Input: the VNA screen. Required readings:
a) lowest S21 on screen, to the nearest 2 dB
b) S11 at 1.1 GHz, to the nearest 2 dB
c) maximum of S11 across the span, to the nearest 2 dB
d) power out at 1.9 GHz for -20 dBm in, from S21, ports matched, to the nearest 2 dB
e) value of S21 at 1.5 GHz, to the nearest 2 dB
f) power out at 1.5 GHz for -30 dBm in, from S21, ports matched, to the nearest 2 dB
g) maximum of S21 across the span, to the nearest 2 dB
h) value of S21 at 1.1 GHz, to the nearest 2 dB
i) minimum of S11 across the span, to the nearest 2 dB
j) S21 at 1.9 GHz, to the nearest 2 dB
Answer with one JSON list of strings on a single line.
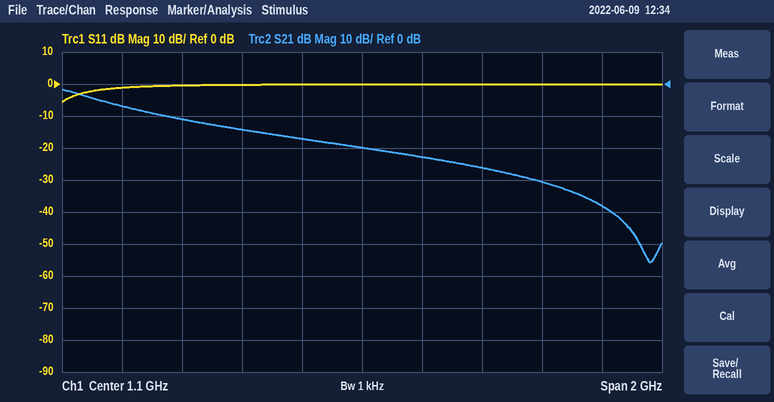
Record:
["-56 dB", "0 dB", "0 dB", "-58 dBm", "-26 dB", "-56 dBm", "-2 dB", "-20 dB", "-6 dB", "-38 dB"]
